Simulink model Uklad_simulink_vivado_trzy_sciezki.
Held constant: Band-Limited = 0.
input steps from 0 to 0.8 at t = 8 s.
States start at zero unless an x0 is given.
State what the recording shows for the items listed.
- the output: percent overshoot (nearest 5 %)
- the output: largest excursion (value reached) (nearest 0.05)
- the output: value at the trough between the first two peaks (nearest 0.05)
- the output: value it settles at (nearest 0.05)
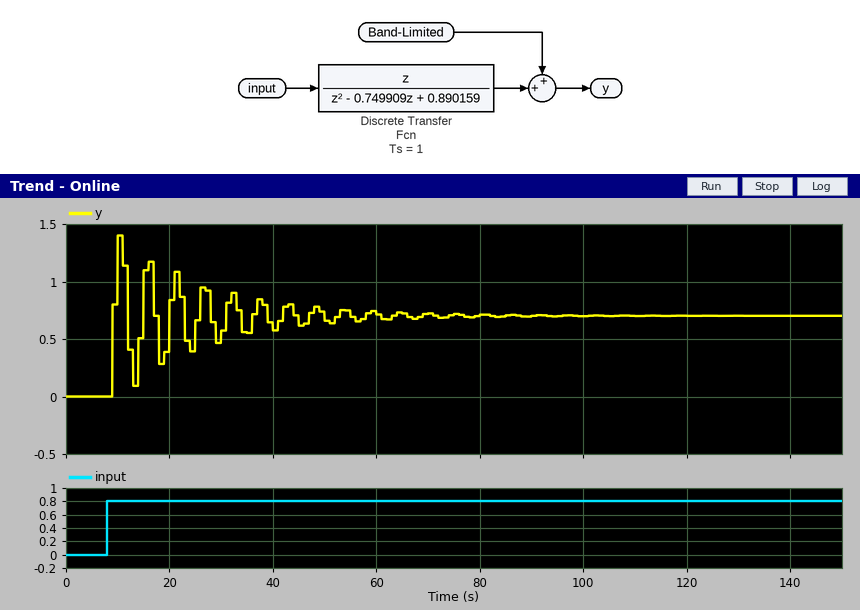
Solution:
100 %
1.40
0.10
0.70
